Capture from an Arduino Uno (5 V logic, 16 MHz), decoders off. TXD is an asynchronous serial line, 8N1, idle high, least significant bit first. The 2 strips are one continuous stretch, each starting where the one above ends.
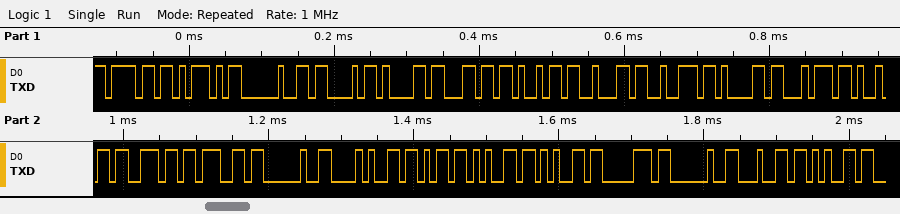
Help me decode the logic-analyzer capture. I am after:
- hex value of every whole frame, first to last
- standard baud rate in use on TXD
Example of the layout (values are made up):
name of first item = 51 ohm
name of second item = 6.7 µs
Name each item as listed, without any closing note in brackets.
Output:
hex value of every whole frame, first to last = 6F 5D 20 43 61 6C 69 62 72 61 74 69 6E 67 20 28 6B 65 65 70 20 64 65
standard baud rate in use on TXD = 115200 baud
